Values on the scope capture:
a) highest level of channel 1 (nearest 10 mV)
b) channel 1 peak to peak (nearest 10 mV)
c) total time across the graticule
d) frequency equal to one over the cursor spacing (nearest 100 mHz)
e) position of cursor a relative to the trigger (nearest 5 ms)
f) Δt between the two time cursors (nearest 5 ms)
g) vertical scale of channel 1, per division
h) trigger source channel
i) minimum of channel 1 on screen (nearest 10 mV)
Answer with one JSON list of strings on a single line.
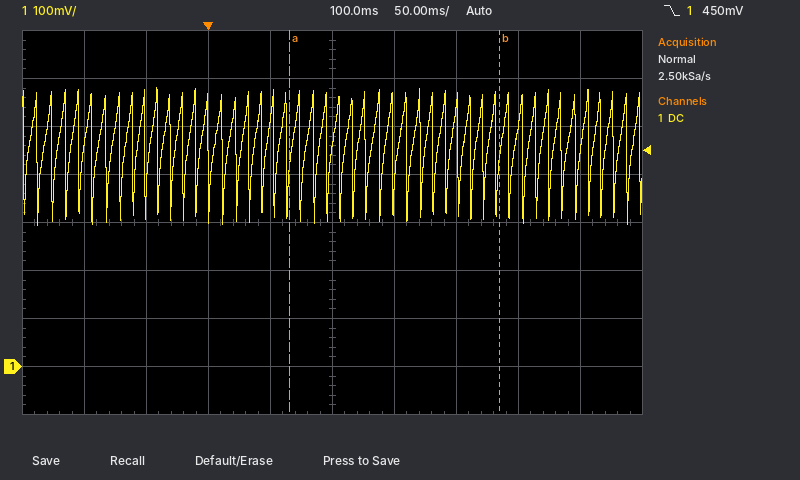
["580 mV", "290 mV", "500 ms", "5.9 Hz", "+65 ms", "170 ms", "100 mV", "channel 1", "290 mV"]
